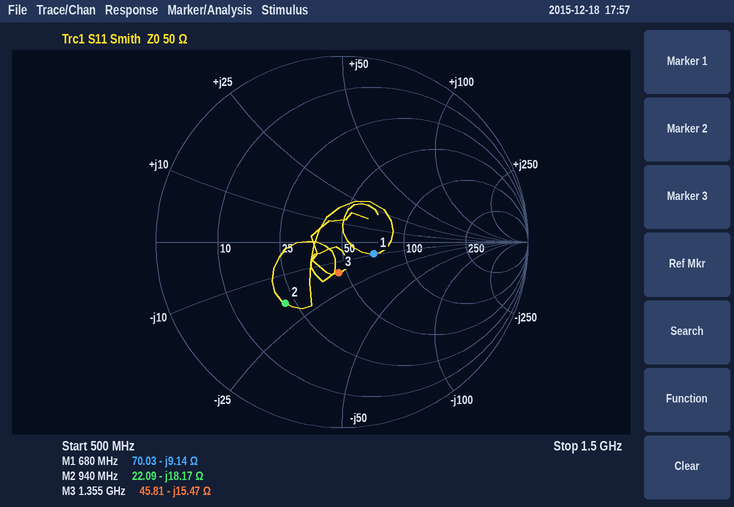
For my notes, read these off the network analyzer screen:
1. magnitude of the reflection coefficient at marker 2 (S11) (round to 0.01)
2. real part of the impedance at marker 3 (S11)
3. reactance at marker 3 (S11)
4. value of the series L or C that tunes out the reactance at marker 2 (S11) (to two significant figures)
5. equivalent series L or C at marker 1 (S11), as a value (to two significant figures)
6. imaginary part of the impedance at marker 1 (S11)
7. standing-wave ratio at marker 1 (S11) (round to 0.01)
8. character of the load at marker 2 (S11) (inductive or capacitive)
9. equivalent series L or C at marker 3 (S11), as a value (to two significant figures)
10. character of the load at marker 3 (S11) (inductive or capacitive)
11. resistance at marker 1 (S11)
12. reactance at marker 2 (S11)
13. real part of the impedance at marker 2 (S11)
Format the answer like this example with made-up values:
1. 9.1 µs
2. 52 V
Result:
1. 0.45
2. 45.81 Ω
3. -15.47 Ω
4. 3.1 nH
5. 26 pF
6. -9.14 Ω
7. 1.45
8. capacitive
9. 7.6 pF
10. capacitive
11. 70.03 Ω
12. -18.17 Ω
13. 22.09 Ω
